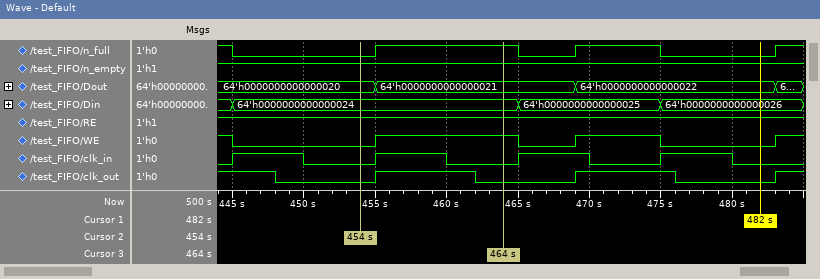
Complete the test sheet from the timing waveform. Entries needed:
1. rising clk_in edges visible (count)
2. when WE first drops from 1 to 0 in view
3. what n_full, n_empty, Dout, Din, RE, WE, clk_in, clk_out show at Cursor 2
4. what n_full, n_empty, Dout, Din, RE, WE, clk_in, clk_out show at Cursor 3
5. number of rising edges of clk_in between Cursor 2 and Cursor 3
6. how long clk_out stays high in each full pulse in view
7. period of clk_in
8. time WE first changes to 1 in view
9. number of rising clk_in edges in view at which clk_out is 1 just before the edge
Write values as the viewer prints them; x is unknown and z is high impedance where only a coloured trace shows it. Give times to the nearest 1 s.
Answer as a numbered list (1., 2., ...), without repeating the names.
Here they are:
1. 4
2. 445 s
3. n_full=0, n_empty=1, Dout=64'h0000000000000020, Din=64'h0000000000000024, RE=1, WE=0, clk_in=0, clk_out=0
4. n_full=1, n_empty=1, Dout=64'h0000000000000021, Din=64'h0000000000000024, RE=1, WE=1, clk_in=0, clk_out=0
5. 1
6. 7 s, 7 s
7. 10 s
8. 455 s
9. 2
